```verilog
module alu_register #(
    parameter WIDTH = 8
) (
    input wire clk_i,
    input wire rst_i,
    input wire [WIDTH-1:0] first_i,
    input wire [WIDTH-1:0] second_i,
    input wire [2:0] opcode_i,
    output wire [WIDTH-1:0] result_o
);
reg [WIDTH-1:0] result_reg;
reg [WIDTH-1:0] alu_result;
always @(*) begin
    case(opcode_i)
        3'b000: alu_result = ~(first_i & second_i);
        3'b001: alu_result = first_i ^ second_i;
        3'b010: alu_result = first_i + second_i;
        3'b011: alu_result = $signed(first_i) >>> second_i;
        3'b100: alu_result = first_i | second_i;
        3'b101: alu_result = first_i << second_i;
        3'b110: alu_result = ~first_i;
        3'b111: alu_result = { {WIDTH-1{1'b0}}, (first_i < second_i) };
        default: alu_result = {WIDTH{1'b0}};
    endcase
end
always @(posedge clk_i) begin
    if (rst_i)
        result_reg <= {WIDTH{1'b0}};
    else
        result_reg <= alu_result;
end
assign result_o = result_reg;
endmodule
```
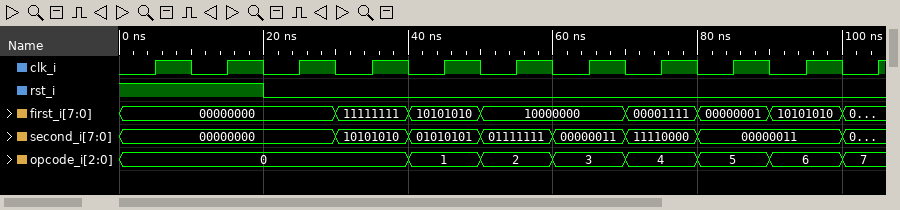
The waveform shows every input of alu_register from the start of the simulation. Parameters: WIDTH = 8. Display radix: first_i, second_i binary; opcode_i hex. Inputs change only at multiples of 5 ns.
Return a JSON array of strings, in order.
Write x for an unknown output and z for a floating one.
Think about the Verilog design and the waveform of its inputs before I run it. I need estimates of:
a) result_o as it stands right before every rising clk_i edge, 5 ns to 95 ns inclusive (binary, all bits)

["x, 00000000, 00000000, 11111111, 01010101, 11111111, 11111111, 11110000, 11111111, 00001000"]
